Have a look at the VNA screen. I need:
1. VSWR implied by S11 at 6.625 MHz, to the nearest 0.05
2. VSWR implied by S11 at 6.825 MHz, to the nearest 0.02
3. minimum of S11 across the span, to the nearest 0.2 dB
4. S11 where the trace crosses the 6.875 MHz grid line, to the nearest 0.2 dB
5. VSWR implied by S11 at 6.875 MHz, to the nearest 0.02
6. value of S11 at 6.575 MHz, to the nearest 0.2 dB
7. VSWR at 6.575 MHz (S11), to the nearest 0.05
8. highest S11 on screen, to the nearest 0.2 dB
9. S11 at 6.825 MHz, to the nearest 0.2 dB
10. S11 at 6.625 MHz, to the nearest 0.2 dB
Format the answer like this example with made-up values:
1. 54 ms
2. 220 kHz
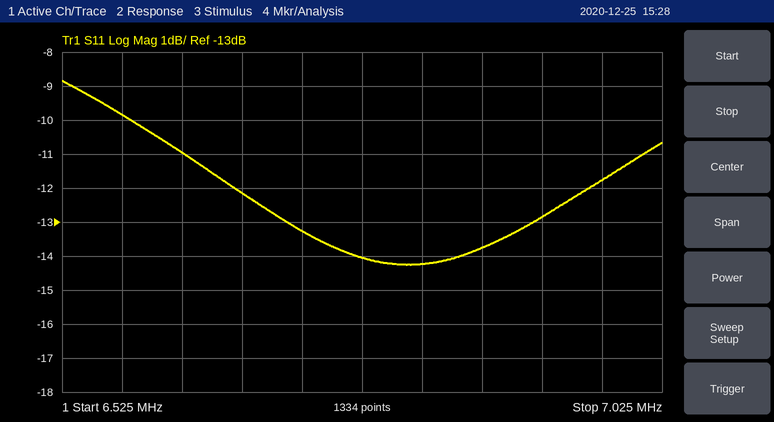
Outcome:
1. 1.80
2. 1.48
3. -14.2 dB
4. -13.8 dB
5. 1.52
6. -9.8 dB
7. 1.95
8. -8.8 dB
9. -14.2 dB
10. -11.0 dB
